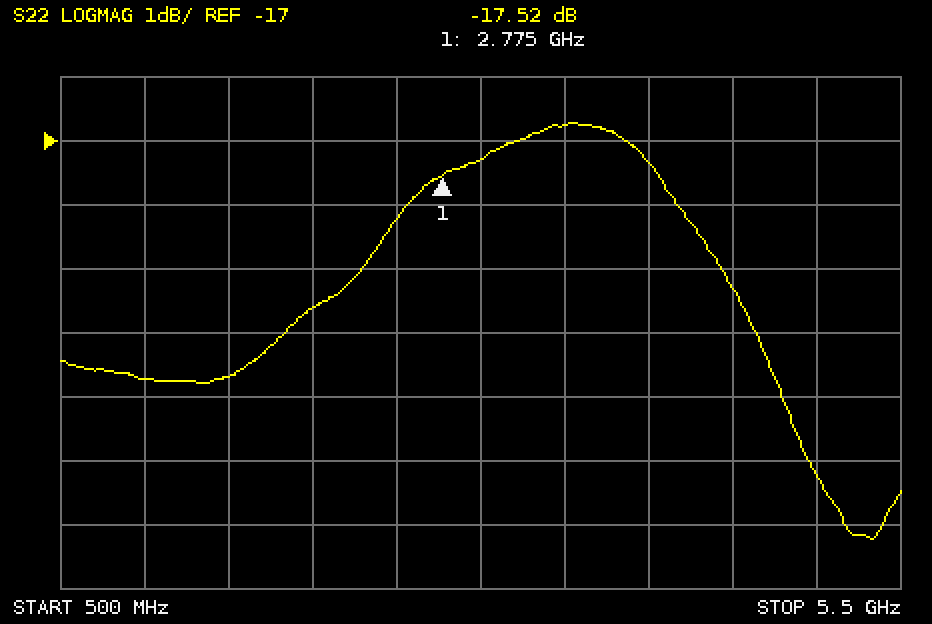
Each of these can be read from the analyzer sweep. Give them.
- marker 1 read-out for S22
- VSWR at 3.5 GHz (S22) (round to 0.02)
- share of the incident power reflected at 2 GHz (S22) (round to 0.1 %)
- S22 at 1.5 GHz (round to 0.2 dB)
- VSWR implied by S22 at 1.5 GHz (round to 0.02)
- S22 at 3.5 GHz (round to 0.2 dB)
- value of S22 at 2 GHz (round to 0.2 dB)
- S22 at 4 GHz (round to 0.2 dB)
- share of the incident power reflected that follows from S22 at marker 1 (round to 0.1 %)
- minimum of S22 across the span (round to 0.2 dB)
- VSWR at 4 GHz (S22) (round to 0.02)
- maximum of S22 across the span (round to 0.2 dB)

-17.52 dB
1.34
1.1 %
-20.6 dB
1.20
-16.8 dB
-19.6 dB
-17.4 dB
1.8 %
-23.2 dB
1.32
-16.8 dB
